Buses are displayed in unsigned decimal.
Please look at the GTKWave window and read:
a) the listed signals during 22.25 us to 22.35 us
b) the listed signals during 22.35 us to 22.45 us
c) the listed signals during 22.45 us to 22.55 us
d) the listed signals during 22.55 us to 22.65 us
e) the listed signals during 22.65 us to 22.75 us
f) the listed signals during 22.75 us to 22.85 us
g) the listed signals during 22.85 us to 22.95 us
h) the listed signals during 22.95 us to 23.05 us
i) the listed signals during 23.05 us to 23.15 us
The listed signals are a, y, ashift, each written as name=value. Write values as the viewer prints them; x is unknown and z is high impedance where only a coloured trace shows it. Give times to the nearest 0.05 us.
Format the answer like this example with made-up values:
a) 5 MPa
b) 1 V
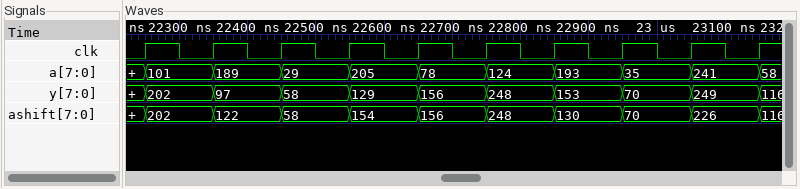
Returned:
a) a=101, y=202, ashift=202
b) a=189, y=97, ashift=122
c) a=29, y=58, ashift=58
d) a=205, y=129, ashift=154
e) a=78, y=156, ashift=156
f) a=124, y=248, ashift=248
g) a=193, y=153, ashift=130
h) a=35, y=70, ashift=70
i) a=241, y=249, ashift=226
